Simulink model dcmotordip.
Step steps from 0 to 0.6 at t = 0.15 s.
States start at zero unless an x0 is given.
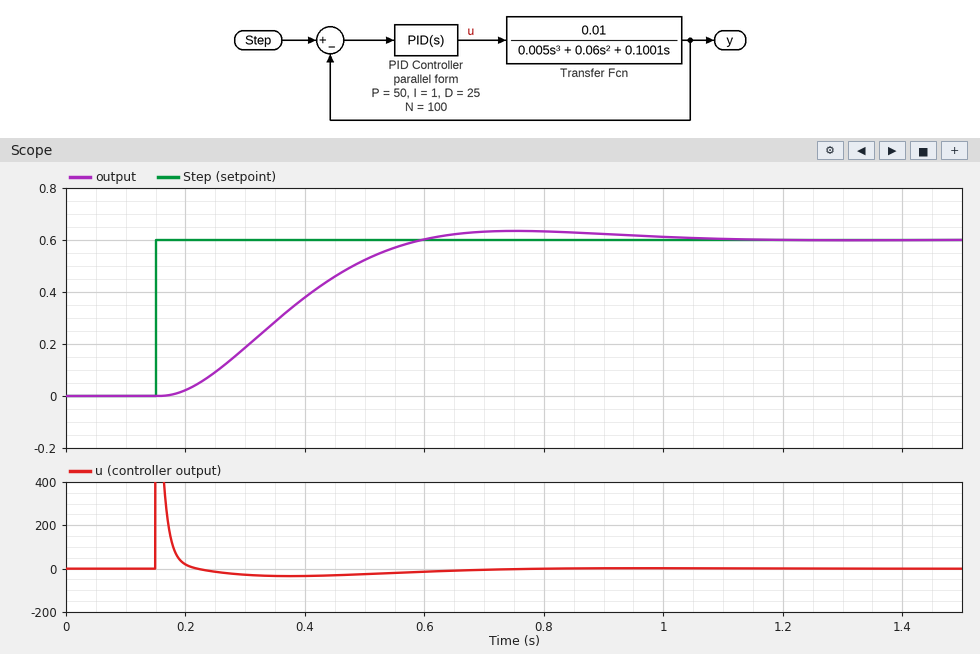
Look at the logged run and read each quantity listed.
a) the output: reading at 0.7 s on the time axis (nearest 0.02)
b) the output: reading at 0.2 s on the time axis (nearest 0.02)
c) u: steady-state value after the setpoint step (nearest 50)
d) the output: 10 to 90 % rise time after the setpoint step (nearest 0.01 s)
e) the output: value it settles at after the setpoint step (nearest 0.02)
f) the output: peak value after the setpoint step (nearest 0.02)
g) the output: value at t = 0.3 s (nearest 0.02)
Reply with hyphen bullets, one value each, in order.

- 0.64
- 0.02
- 0
- 0.29 s
- 0.60
- 0.64
- 0.18
